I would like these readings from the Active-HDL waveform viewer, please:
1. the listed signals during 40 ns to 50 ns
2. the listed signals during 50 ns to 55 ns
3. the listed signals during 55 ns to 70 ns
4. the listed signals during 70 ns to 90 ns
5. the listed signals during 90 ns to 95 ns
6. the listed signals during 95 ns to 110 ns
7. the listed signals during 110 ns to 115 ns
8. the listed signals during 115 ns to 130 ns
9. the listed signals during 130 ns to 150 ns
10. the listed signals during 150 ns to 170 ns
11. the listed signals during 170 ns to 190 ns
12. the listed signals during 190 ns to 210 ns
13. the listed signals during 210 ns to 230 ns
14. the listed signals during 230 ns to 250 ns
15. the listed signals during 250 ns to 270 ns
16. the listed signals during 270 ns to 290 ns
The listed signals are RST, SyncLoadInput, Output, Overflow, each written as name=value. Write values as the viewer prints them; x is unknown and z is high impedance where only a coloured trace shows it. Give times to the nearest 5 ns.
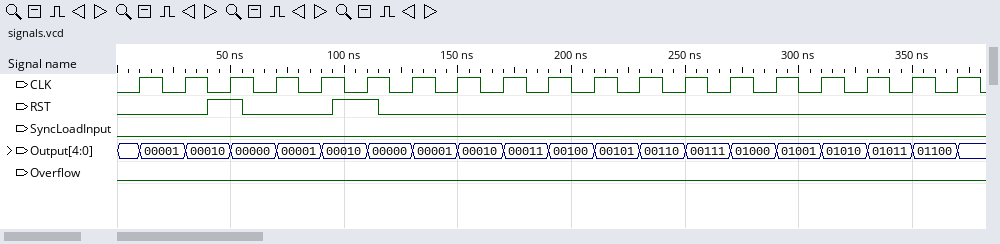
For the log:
RST=1, SyncLoadInput=0, Output=00010, Overflow=0
RST=1, SyncLoadInput=0, Output=00000, Overflow=0
RST=0, SyncLoadInput=0, Output=00000, Overflow=0
RST=0, SyncLoadInput=0, Output=00001, Overflow=0
RST=0, SyncLoadInput=0, Output=00010, Overflow=0
RST=1, SyncLoadInput=0, Output=00010, Overflow=0
RST=1, SyncLoadInput=0, Output=00000, Overflow=0
RST=0, SyncLoadInput=0, Output=00000, Overflow=0
RST=0, SyncLoadInput=0, Output=00001, Overflow=0
RST=0, SyncLoadInput=0, Output=00010, Overflow=0
RST=0, SyncLoadInput=0, Output=00011, Overflow=0
RST=0, SyncLoadInput=0, Output=00100, Overflow=0
RST=0, SyncLoadInput=0, Output=00101, Overflow=0
RST=0, SyncLoadInput=0, Output=00110, Overflow=0
RST=0, SyncLoadInput=0, Output=00111, Overflow=0
RST=0, SyncLoadInput=0, Output=01000, Overflow=0
